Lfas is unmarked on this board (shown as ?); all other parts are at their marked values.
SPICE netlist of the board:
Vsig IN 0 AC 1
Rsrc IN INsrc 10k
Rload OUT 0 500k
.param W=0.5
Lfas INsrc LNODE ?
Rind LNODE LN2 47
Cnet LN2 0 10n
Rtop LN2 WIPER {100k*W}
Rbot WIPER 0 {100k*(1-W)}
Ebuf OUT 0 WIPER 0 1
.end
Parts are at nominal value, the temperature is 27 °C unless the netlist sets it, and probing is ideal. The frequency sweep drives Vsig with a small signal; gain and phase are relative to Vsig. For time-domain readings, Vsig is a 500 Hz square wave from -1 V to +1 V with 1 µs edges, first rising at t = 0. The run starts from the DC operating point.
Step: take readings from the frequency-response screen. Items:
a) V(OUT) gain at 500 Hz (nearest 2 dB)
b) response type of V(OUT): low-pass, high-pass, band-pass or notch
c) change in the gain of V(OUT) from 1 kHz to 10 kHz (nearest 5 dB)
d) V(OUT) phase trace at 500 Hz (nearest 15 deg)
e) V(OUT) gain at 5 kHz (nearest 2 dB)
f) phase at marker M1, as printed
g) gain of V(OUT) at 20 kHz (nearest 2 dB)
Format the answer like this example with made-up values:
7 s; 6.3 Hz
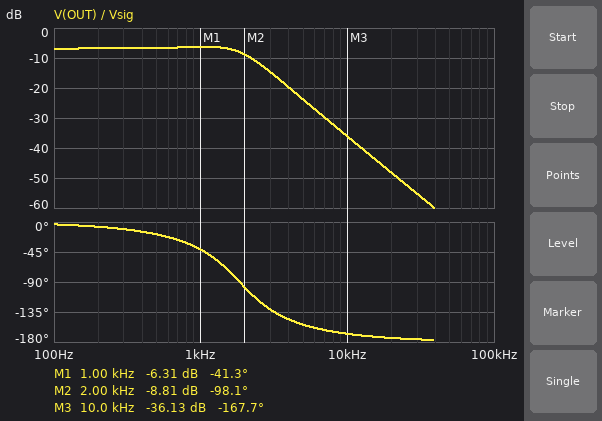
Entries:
-6 dB; low-pass; -30 dB; -15 deg; -24 dB; -41.3 deg; -48 dB
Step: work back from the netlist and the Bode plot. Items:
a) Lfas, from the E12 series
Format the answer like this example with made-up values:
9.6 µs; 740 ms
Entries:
820 mH
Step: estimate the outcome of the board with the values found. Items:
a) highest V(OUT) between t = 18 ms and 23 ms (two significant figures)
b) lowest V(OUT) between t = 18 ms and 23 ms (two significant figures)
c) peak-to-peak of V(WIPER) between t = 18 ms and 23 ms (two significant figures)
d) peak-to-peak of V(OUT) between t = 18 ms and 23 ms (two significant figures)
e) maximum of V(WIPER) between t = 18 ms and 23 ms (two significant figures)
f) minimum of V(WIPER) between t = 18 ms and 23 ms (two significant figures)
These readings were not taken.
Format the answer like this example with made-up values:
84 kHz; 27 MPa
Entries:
560 mV; -560 mV; 1.1 V; 1.1 V; 560 mV; -560 mV
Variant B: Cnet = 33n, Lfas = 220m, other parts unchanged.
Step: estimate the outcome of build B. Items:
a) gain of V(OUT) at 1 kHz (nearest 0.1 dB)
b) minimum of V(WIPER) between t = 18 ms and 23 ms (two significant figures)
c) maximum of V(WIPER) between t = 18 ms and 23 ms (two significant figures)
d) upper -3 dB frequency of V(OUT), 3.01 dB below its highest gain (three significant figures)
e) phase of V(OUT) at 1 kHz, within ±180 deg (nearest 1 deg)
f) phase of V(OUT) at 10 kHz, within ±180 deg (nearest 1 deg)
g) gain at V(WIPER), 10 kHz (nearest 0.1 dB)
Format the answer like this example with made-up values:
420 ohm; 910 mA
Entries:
-13.1 dB; -430 mV; 430 mV; 565 Hz; -69 deg; -143 deg; -36.8 dB
